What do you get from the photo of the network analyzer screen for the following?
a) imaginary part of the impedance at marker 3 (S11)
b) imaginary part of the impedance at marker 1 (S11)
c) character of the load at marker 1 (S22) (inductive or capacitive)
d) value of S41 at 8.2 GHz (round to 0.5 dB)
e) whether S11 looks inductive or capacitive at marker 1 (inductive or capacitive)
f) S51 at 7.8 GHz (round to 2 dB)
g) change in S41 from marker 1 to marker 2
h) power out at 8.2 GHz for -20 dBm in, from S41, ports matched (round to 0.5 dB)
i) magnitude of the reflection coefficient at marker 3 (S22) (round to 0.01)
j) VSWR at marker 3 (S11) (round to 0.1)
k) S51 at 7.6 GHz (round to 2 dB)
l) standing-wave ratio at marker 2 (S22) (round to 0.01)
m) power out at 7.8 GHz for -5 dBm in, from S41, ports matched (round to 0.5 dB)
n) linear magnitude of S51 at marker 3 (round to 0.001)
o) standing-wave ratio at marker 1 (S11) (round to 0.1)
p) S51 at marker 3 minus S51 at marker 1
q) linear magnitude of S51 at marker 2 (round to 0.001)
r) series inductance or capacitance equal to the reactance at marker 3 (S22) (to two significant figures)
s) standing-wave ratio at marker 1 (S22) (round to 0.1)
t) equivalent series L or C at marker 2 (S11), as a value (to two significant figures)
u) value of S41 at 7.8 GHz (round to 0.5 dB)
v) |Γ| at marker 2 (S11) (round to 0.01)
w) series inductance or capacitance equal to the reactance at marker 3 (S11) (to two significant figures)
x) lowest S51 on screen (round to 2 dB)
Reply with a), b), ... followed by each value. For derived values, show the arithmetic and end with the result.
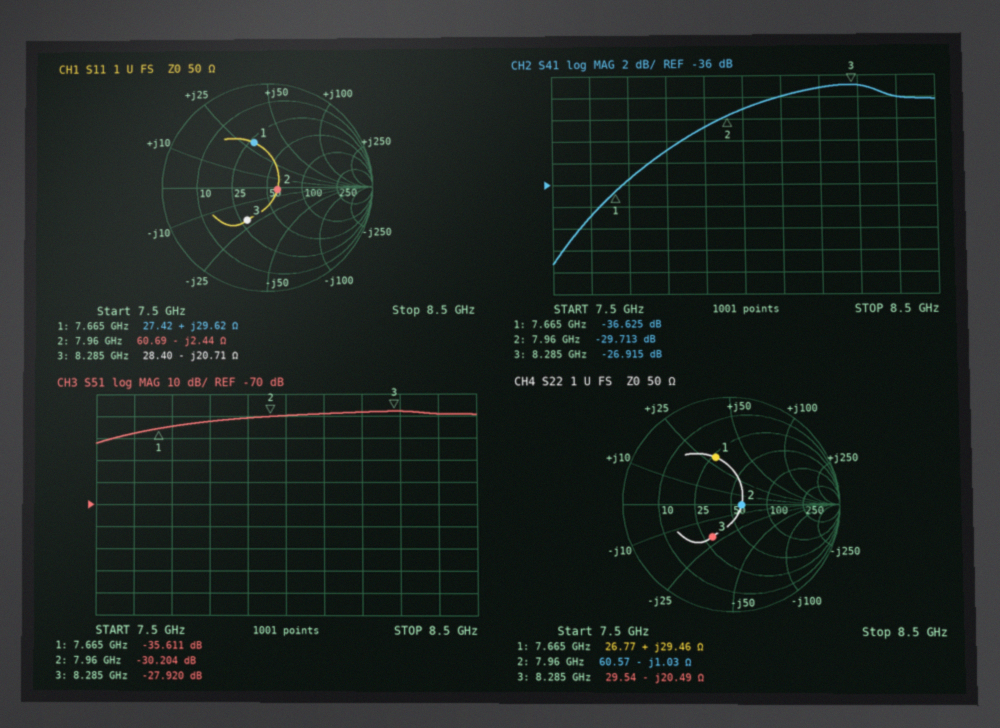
a) -20.71 Ω
b) +29.62 Ω
c) inductive
d) -27.0 dB
e) inductive
f) -32 dB
g) -29.713 − (-36.625) = 6.912 dB
h) -20 dBm + (-27.0 dB) = -47.0 dBm
i) 0.35
j) 2.2
k) -38 dB
l) 1.21
m) -5 dBm + (-33.0 dB) = -38.0 dBm
n) 10^(-27.92/20) ≈ 0.040
o) 2.6
p) -27.92 − (-35.611) = 7.691 dB
q) 10^(-30.204/20) ≈ 0.031
r) C = 1/(2π × 8.285 GHz × 20.49 Ω) ≈ 938 fF, so 940 fF to two significant figures
s) 2.7
t) C = 1/(2π × 7.96 GHz × 2.44 Ω) ≈ 8.2 pF
u) -33.0 dB
v) 0.10
w) C = 1/(2π × 8.285 GHz × 20.71 Ω) ≈ 928 fF, so 930 fF to two significant figures
x) -42 dB
